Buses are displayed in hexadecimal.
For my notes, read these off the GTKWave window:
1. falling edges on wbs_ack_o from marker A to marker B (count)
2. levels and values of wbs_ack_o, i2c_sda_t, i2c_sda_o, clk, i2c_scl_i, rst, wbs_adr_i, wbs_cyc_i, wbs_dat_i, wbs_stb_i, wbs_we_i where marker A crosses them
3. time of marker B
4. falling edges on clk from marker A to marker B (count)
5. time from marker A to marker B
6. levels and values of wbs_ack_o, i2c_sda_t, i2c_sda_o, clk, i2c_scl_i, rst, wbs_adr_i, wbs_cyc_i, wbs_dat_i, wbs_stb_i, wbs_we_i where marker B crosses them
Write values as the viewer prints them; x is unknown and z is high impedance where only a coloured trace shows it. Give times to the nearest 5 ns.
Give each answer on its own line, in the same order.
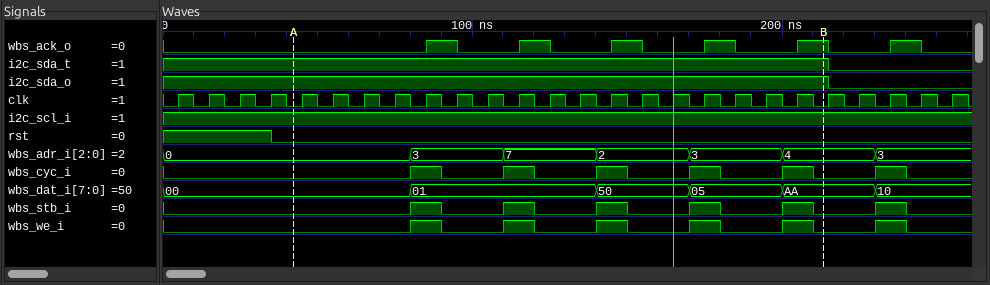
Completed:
4
wbs_ack_o=0, i2c_sda_t=1, i2c_sda_o=1, clk=0, i2c_scl_i=1, rst=0, wbs_adr_i=0, wbs_cyc_i=0, wbs_dat_i=00, wbs_stb_i=0, wbs_we_i=0
215 ns
17
170 ns
wbs_ack_o=1, i2c_sda_t=1, i2c_sda_o=1, clk=0, i2c_scl_i=1, rst=0, wbs_adr_i=4, wbs_cyc_i=0, wbs_dat_i=AA, wbs_stb_i=0, wbs_we_i=0
